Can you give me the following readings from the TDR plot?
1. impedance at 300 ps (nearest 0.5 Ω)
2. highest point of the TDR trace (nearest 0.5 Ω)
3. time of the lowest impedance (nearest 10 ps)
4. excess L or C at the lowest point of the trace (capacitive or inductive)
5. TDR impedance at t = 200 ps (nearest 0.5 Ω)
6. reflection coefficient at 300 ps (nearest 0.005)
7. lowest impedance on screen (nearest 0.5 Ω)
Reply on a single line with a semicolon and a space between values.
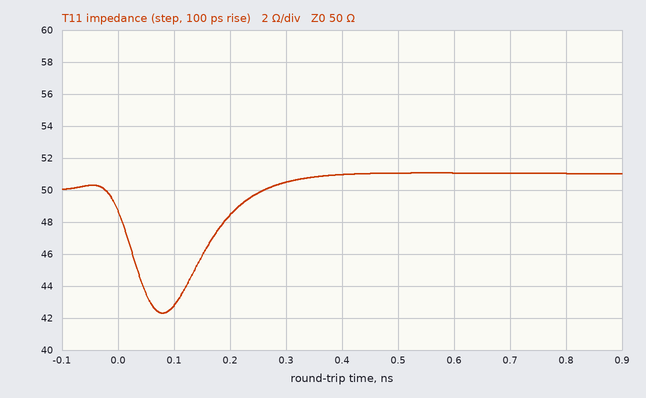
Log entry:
50.5 Ω; 51.0 Ω; 80 ps; capacitive; 48.5 Ω; +0.005; 42.5 Ω
